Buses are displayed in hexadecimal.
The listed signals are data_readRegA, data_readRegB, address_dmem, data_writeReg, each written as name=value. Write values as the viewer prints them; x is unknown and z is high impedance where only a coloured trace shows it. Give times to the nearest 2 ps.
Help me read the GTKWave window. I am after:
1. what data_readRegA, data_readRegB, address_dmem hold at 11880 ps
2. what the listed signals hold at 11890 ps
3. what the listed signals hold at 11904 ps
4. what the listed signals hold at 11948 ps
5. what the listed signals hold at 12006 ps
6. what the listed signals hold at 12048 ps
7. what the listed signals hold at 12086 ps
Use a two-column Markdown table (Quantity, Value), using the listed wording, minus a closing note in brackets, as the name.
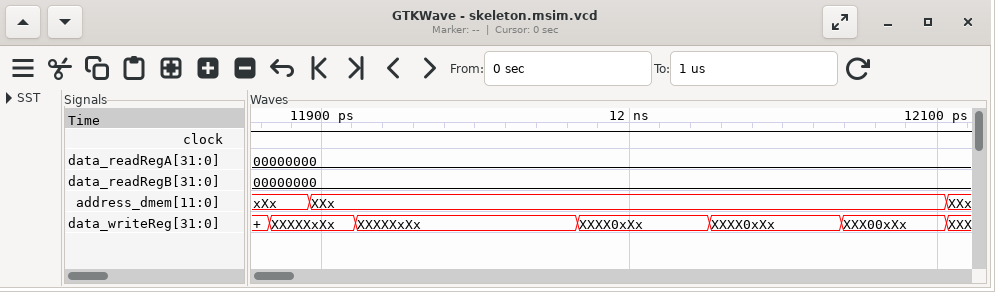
| Quantity | Value |
|---|---|
| what data_readRegA, data_readRegB, address_dmem hold at 11880 ps | data_readRegA=00000000, data_readRegB=00000000, address_dmem=xXx |
| what the listed signals hold at 11890 ps | data_readRegA=00000000, data_readRegB=00000000, address_dmem=xXx, data_writeReg=XXXXXxXx |
| what the listed signals hold at 11904 ps | data_readRegA=00000000, data_readRegB=00000000, address_dmem=XXx, data_writeReg=XXXXXxXx |
| what the listed signals hold at 11948 ps | data_readRegA=00000000, data_readRegB=00000000, address_dmem=XXx, data_writeReg=XXXXXxXx |
| what the listed signals hold at 12006 ps | data_readRegA=00000000, data_readRegB=00000000, address_dmem=XXx, data_writeReg=XXXX0xXx |
| what the listed signals hold at 12048 ps | data_readRegA=00000000, data_readRegB=00000000, address_dmem=XXx, data_writeReg=XXXX0xXx |
| what the listed signals hold at 12086 ps | data_readRegA=00000000, data_readRegB=00000000, address_dmem=XXx, data_writeReg=XXX00xXx |
